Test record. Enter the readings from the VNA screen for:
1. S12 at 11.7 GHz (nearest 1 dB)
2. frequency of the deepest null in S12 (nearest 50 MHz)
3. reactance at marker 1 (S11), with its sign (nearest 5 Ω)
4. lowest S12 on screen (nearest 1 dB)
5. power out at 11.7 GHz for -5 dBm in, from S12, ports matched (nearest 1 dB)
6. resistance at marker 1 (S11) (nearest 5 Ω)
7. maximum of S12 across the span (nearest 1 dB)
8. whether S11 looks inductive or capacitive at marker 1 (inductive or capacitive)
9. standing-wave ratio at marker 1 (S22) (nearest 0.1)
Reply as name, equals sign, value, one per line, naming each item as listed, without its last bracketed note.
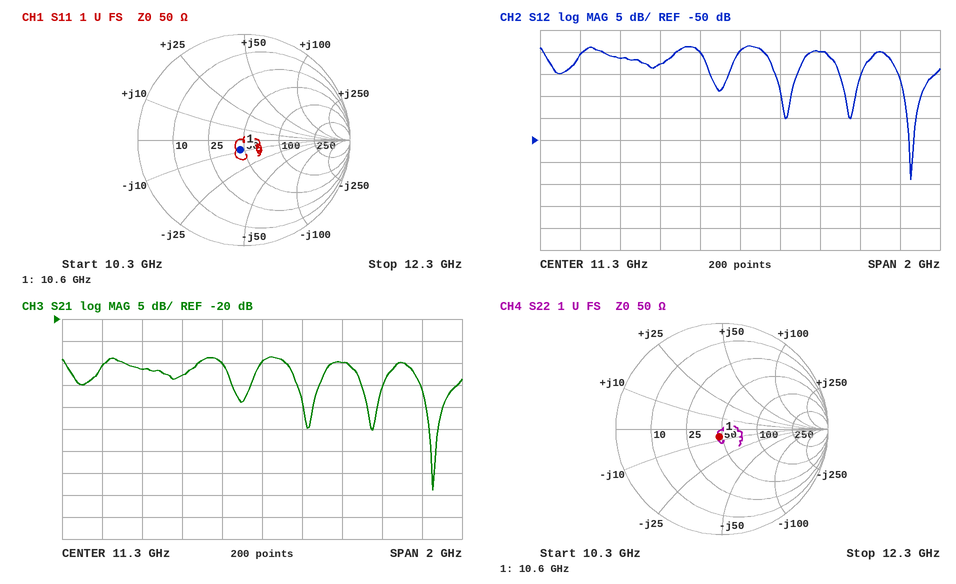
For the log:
S12 at 11.7 GHz = -30 dB
frequency of the deepest null in S12 = 12.15 GHz
reactance at marker 1 (S11), with its sign = -10 Ω
lowest S12 on screen = -59 dB
power out at 11.7 GHz for -5 dBm in, from S12, ports matched = -35 dBm
resistance at marker 1 (S11) = 45 Ω
maximum of S12 across the span = -29 dB
whether S11 looks inductive or capacitive at marker 1 = capacitive
standing-wave ratio at marker 1 (S22) = 1.2
